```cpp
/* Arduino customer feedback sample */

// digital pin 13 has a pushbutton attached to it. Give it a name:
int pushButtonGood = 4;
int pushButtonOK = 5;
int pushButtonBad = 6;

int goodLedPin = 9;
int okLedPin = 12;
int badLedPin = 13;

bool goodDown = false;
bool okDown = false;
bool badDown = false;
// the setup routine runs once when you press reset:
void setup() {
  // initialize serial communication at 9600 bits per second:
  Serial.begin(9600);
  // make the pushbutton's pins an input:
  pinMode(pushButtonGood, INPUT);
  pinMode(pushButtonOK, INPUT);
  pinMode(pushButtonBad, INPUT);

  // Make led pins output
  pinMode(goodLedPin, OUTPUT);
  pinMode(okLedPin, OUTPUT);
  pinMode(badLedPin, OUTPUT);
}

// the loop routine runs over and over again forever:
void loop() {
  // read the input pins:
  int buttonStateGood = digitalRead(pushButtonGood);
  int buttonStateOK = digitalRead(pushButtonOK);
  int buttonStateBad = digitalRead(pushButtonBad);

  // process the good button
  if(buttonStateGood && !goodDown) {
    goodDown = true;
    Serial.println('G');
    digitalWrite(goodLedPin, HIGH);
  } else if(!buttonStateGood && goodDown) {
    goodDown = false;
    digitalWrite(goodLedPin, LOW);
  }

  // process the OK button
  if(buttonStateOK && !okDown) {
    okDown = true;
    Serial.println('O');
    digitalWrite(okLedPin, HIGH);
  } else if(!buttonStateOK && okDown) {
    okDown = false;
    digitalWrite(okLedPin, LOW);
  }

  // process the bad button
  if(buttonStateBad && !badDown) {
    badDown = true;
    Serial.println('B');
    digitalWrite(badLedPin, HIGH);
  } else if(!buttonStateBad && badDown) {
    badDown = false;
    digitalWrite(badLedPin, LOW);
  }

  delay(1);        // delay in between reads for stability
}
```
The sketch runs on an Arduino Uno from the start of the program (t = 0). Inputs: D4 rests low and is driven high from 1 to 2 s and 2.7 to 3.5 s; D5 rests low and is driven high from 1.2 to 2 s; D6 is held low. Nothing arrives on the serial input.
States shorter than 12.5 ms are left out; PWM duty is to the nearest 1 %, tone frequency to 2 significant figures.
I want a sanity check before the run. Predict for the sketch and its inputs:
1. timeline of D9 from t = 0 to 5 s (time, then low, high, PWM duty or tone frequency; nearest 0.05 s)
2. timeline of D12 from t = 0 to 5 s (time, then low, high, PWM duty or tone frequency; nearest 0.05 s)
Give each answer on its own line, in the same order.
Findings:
0 s low; 1 s high; 2 s low; 2.7 s high; 3.5 s low
0 s low; 1.2 s high; 2 s low
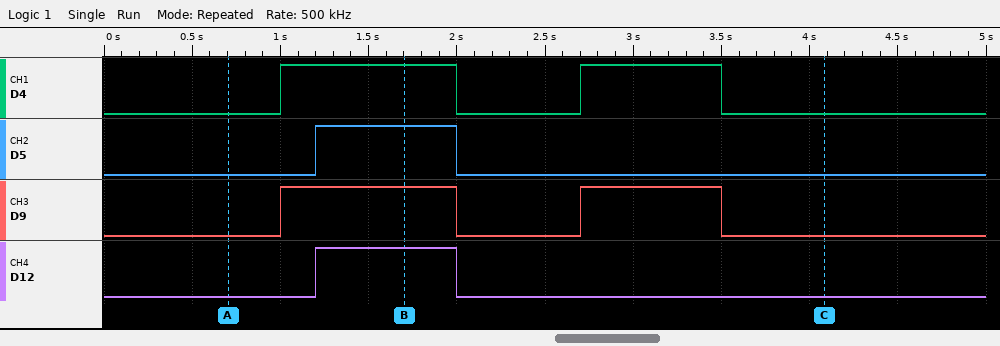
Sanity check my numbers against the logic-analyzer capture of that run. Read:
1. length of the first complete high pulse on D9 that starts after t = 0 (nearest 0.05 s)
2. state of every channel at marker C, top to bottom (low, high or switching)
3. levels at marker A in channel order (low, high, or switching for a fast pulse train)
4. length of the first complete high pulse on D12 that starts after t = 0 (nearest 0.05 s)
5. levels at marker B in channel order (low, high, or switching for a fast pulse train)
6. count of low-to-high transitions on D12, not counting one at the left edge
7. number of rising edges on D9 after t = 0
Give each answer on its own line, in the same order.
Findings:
1.00 s
D4 low, D5 low, D9 low, D12 low
D4 low, D5 low, D9 low, D12 low
0.80 s
D4 high, D5 high, D9 high, D12 high
1
2
